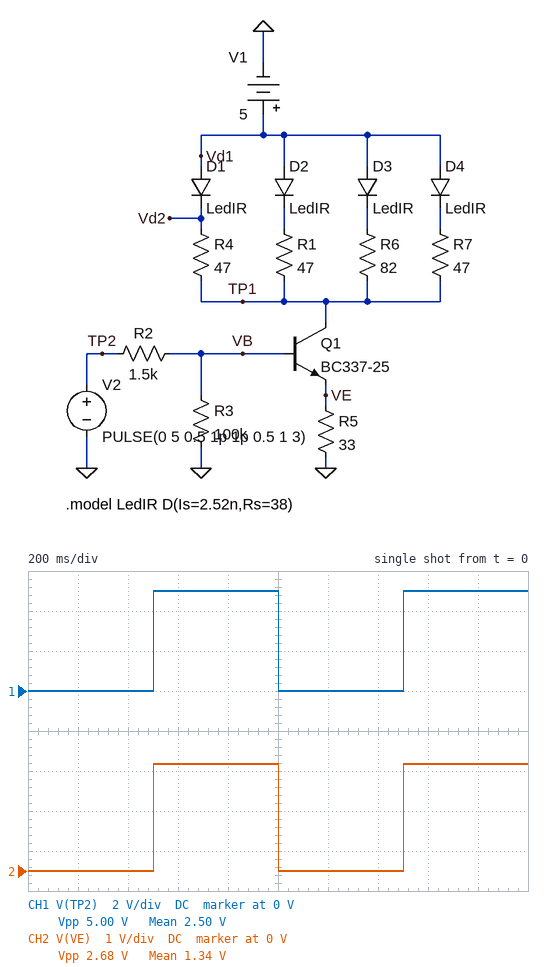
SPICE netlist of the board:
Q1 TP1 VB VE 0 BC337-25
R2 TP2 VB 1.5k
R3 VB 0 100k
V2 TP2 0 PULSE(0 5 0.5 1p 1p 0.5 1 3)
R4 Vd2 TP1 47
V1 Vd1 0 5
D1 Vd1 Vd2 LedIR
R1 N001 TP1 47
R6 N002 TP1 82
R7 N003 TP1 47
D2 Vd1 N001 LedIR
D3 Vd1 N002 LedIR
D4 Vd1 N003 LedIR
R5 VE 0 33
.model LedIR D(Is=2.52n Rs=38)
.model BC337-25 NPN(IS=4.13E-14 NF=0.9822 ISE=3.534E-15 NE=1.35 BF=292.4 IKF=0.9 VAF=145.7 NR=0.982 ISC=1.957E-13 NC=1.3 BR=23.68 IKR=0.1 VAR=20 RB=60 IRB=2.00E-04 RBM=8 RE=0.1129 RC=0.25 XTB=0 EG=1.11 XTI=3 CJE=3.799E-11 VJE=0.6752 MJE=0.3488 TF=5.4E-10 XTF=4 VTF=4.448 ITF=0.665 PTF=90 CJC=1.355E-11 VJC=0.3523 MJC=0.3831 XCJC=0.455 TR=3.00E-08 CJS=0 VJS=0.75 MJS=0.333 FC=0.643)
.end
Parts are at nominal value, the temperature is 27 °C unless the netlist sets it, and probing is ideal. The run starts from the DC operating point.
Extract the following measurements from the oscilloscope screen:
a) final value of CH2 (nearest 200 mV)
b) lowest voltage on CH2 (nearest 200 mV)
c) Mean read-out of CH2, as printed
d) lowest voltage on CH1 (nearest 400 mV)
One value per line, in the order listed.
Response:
2.6 V
0 V
1.34 V
0 V
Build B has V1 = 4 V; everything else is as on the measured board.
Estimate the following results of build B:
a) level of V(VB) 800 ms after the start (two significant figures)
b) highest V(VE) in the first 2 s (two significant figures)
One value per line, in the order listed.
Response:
2.9 V
2.1 V
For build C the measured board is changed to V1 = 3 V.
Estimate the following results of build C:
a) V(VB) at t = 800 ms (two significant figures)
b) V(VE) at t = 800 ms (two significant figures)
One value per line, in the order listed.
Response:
2.3 V
1.5 V
